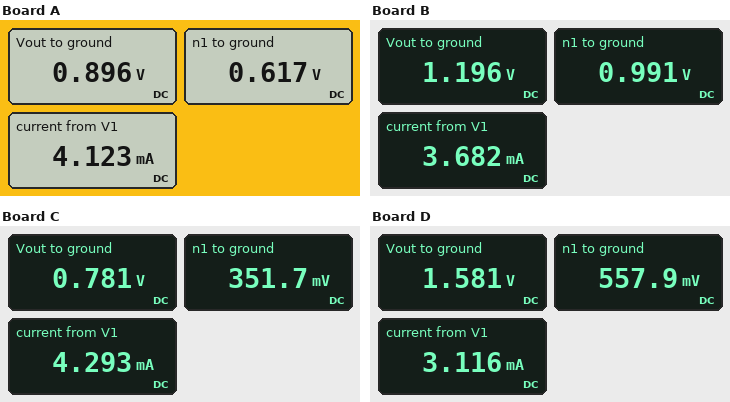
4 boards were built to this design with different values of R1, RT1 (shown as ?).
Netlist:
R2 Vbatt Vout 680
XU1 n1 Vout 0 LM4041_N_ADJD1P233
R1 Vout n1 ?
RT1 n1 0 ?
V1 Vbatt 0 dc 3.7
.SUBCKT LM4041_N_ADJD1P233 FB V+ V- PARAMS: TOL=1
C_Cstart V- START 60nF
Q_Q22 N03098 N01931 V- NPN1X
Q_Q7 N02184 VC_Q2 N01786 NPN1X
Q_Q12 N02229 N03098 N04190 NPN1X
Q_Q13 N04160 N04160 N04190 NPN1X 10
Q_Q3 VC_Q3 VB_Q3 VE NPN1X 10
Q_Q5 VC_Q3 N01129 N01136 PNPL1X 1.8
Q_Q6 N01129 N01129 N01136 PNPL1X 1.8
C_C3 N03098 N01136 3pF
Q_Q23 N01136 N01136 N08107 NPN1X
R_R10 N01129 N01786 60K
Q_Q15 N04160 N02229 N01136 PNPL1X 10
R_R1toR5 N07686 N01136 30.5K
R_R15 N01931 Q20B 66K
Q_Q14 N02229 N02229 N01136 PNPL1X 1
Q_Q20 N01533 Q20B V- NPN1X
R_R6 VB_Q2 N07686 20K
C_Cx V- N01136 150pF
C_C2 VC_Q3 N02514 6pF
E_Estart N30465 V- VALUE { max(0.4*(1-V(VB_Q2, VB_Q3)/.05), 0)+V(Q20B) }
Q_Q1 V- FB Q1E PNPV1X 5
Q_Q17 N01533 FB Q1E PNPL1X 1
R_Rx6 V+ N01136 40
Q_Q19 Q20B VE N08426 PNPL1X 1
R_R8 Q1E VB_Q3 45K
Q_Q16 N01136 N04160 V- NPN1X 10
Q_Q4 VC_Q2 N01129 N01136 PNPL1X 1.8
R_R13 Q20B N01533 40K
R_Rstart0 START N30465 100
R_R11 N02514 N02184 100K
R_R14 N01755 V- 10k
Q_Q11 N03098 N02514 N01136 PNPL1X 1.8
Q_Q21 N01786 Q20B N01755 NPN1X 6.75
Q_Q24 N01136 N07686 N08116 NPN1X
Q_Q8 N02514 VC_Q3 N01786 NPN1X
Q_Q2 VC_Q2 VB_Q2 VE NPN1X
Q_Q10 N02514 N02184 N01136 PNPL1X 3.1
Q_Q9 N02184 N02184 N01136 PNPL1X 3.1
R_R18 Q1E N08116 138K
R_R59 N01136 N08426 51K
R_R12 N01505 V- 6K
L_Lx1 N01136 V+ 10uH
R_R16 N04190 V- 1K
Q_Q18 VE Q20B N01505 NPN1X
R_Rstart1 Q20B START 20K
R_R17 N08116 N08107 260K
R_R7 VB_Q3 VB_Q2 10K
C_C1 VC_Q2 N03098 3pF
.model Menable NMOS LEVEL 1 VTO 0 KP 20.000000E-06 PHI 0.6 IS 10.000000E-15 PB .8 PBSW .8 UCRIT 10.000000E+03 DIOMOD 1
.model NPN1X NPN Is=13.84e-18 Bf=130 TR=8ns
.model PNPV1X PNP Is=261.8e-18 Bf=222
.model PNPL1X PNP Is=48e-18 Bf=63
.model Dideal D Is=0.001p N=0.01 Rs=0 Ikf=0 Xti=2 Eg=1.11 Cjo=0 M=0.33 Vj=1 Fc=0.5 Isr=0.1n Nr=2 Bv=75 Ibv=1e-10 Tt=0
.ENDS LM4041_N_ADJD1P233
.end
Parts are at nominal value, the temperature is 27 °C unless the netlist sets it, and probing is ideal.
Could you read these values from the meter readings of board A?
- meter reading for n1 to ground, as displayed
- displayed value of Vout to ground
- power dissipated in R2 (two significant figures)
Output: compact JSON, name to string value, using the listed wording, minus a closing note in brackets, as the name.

{"meter reading for n1 to ground, as displayed": "0.617 V", "displayed value of Vout to ground": "0.896 V", "power dissipated in R2": "12 mW"}
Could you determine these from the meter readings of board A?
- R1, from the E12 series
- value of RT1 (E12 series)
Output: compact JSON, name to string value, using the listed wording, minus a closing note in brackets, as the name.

{"R1, from the E12 series": "68 Ω", "value of RT1": "150 Ω"}
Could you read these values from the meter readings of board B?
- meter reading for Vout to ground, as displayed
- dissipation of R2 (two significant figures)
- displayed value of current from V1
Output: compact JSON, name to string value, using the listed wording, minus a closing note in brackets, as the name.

{"meter reading for Vout to ground, as displayed": "1.196 V", "dissipation of R2": "9.2 mW", "displayed value of current from V1": "3.682 mA"}
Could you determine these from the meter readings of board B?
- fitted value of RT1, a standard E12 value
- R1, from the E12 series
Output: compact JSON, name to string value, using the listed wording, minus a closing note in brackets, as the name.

{"fitted value of RT1, a standard E12 value": "270 Ω", "R1, from the E12 series": "56 Ω"}
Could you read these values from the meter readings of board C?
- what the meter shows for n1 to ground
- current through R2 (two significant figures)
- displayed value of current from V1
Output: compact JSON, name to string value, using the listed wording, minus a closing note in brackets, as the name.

{"what the meter shows for n1 to ground": "351.7 mV", "current through R2": "4.3 mA", "displayed value of current from V1": "4.293 mA"}
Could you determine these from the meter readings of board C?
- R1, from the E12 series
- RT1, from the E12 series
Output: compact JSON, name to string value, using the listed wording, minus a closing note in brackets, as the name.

{"R1, from the E12 series": "100 Ω", "RT1, from the E12 series": "82 Ω"}
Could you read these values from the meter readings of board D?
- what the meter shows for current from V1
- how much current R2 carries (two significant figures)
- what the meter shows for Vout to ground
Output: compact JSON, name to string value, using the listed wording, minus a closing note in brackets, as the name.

{"what the meter shows for current from V1": "3.116 mA", "how much current R2 carries": "3.1 mA", "what the meter shows for Vout to ground": "1.581 V"}
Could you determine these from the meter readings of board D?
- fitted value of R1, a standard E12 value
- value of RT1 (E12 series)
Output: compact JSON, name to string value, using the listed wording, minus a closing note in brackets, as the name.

{"fitted value of R1, a standard E12 value": "330 Ω", "value of RT1": "180 Ω"}
